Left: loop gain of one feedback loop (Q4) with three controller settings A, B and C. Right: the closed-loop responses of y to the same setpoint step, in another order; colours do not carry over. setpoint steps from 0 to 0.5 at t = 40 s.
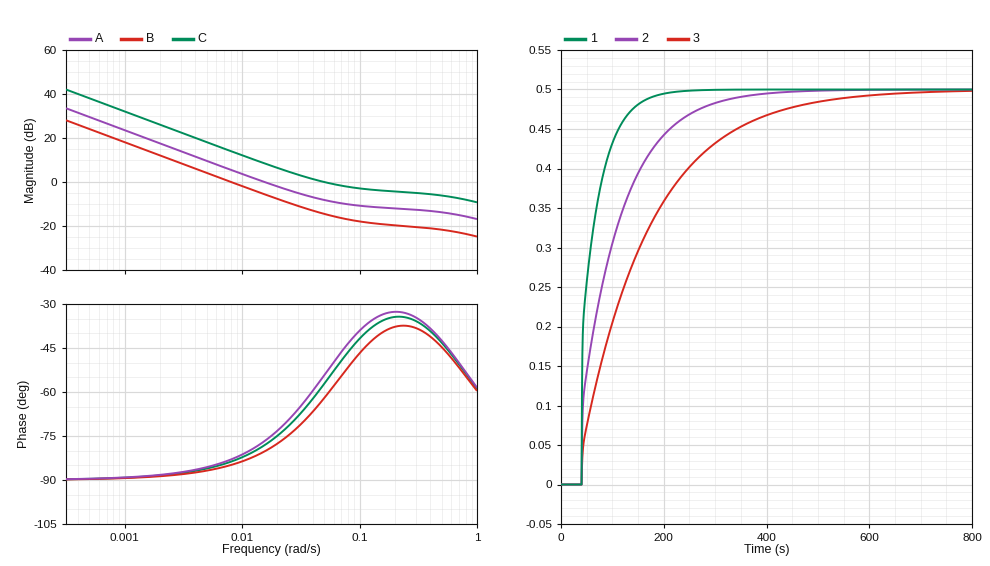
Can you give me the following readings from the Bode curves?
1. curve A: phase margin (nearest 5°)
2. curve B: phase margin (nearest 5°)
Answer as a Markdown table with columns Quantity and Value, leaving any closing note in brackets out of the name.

| Quantity | Value |
|---|---|
| curve A: phase margin | 105° |
| curve B: phase margin | 95° |
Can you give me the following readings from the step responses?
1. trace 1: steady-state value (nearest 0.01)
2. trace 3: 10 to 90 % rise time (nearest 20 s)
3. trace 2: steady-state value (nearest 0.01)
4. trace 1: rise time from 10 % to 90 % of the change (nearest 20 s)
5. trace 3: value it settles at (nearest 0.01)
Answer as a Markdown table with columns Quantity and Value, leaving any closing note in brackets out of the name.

| Quantity | Value |
|---|---|
| trace 1: steady-state value | 0.50 |
| trace 3: 10 to 90 % rise time | 300 s |
| trace 2: steady-state value | 0.50 |
| trace 1: rise time from 10 % to 90 % of the change | 80 s |
| trace 3: value it settles at | 0.50 |
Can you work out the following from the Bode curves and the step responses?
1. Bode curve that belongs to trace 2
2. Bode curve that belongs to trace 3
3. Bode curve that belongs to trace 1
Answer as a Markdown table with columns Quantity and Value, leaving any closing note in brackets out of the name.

| Quantity | Value |
|---|---|
| Bode curve that belongs to trace 2 | A |
| Bode curve that belongs to trace 3 | B |
| Bode curve that belongs to trace 1 | C |
